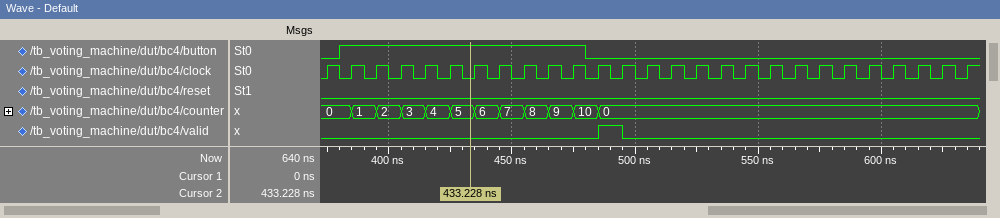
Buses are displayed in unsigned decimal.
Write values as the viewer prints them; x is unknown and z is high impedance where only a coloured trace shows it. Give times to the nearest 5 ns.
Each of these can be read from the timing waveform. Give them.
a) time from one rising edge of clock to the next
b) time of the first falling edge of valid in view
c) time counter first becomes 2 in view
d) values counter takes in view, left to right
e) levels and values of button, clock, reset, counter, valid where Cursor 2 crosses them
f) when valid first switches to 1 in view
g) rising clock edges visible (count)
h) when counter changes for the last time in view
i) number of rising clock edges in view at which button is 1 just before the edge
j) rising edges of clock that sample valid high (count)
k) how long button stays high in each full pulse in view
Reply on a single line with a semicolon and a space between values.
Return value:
10 ns; 495 ns; 395 ns; 0, 1, 2, 3, 4, 5, 6, 7, 8, 9, 10, 0; button=1, clock=0, reset=0, counter=5, valid=0; 485 ns; 27; 485 ns; 10; 1; 100 ns
